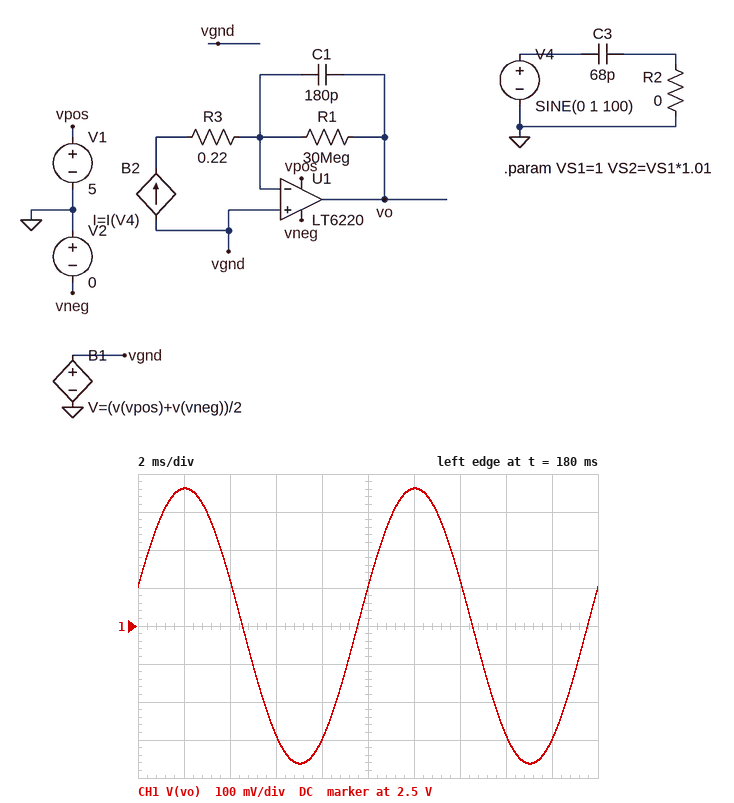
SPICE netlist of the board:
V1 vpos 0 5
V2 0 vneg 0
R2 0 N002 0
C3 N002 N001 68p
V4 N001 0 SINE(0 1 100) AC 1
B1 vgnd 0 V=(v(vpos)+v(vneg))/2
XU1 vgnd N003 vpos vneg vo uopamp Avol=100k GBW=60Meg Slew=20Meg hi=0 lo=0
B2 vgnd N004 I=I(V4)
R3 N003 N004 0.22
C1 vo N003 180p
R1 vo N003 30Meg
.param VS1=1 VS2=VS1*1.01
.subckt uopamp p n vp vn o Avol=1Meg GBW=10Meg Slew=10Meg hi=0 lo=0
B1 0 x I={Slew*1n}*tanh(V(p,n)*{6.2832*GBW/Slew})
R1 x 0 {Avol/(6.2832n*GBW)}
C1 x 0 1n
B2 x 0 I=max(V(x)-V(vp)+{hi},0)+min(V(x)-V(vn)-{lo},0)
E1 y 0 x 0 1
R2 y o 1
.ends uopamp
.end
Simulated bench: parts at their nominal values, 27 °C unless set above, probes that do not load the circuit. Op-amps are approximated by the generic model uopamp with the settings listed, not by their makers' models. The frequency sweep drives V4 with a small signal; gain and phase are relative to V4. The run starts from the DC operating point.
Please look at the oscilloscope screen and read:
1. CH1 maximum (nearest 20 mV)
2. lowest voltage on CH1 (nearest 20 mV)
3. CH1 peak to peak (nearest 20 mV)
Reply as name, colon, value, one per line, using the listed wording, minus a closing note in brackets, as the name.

CH1 maximum: 2.86 V
lowest voltage on CH1: 2.14 V
CH1 peak to peak: 720 mV
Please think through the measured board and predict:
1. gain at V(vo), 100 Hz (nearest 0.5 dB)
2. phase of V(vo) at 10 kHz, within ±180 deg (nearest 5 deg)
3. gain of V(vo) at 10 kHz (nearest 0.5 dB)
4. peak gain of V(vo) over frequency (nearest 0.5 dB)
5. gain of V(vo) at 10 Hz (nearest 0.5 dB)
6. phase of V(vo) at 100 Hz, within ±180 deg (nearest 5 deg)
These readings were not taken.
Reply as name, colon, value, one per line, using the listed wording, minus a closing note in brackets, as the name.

gain at V(vo), 100 Hz: -9.0 dB
phase of V(vo) at 10 kHz, within ±180 deg: 0 deg
gain of V(vo) at 10 kHz: -8.5 dB
peak gain of V(vo) over frequency: -8.5 dB
gain of V(vo) at 10 Hz: -18.5 dB
phase of V(vo) at 100 Hz, within ±180 deg: 15 deg
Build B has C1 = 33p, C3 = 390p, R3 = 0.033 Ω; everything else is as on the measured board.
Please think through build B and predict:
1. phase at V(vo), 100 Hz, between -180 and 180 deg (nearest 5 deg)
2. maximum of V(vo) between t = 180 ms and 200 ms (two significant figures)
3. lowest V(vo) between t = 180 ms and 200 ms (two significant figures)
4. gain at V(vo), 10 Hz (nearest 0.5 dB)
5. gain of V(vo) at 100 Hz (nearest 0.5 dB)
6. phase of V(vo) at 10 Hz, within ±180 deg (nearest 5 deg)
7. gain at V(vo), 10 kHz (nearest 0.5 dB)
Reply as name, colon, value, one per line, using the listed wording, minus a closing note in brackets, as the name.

phase at V(vo), 100 Hz, between -180 and 180 deg: 60 deg
maximum of V(vo) between t = 180 ms and 200 ms: 5.0 V
lowest V(vo) between t = 180 ms and 200 ms: -20 mV
gain at V(vo), 10 Hz: -2.5 dB
gain of V(vo) at 100 Hz: 16.0 dB
phase of V(vo) at 10 Hz, within ±180 deg: 85 deg
gain at V(vo), 10 kHz: 21.5 dB
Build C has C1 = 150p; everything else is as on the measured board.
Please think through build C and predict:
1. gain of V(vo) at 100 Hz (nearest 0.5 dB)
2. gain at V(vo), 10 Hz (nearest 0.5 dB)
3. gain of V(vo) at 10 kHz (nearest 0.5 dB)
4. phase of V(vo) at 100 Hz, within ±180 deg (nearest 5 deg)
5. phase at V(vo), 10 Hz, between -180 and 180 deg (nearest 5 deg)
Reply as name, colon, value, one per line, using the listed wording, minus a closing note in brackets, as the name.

gain of V(vo) at 100 Hz: -7.5 dB
gain at V(vo), 10 Hz: -18.0 dB
gain of V(vo) at 10 kHz: -7.0 dB
phase of V(vo) at 100 Hz, within ±180 deg: 20 deg
phase at V(vo), 10 Hz, between -180 and 180 deg: 75 deg
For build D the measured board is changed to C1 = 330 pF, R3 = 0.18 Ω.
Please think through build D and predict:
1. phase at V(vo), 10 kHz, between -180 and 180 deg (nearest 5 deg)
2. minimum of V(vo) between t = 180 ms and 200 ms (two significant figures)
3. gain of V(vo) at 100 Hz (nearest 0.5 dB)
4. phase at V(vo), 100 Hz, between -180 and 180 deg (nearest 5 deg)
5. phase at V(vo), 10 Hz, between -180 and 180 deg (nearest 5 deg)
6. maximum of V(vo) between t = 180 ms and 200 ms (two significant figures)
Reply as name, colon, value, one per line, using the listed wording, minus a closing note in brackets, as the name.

phase at V(vo), 10 kHz, between -180 and 180 deg: 0 deg
minimum of V(vo) between t = 180 ms and 200 ms: 2.3 V
gain of V(vo) at 100 Hz: -14.0 dB
phase at V(vo), 100 Hz, between -180 and 180 deg: 10 deg
phase at V(vo), 10 Hz, between -180 and 180 deg: 60 deg
maximum of V(vo) between t = 180 ms and 200 ms: 2.7 V
